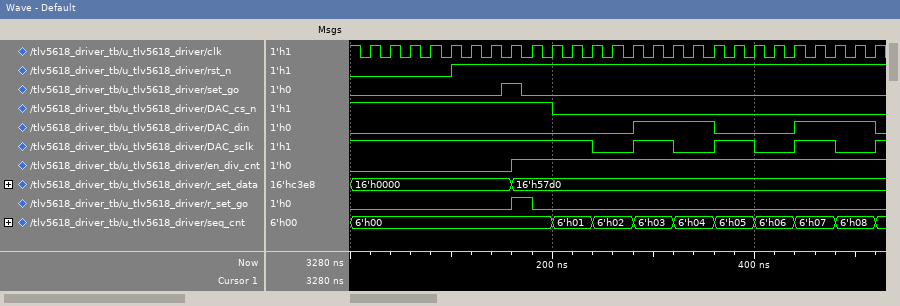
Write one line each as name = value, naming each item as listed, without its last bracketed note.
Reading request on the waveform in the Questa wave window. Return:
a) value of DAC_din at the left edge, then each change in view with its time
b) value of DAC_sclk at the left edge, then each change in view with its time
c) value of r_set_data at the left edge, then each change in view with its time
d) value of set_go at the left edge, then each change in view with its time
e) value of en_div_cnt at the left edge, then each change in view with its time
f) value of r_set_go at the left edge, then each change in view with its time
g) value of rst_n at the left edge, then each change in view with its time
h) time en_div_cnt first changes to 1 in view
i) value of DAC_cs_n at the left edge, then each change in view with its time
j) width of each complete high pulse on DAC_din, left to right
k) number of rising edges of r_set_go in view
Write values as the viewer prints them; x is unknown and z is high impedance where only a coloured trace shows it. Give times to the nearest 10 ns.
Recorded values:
value of DAC_din at the left edge, then each change in view with its time = 0, 1 at 280 ns, 0 at 360 ns, 1 at 440 ns, 0 at 520 ns
value of DAC_sclk at the left edge, then each change in view with its time = 1, 0 at 240 ns, 1 at 280 ns, 0 at 320 ns, 1 at 360 ns, 0 at 400 ns, 1 at 440 ns, 0 at 480 ns, 1 at 520 ns
value of r_set_data at the left edge, then each change in view with its time = 16'h0000, 16'h57d0 at 160 ns
value of set_go at the left edge, then each change in view with its time = 0, 1 at 150 ns, 0 at 170 ns
value of en_div_cnt at the left edge, then each change in view with its time = 0, 1 at 160 ns
value of r_set_go at the left edge, then each change in view with its time = 0, 1 at 160 ns, 0 at 180 ns
value of rst_n at the left edge, then each change in view with its time = 0, 1 at 100 ns
time en_div_cnt first changes to 1 in view = 160 ns
value of DAC_cs_n at the left edge, then each change in view with its time = 1, 0 at 200 ns
width of each complete high pulse on DAC_din, left to right = 80 ns, 80 ns
number of rising edges of r_set_go in view = 1
